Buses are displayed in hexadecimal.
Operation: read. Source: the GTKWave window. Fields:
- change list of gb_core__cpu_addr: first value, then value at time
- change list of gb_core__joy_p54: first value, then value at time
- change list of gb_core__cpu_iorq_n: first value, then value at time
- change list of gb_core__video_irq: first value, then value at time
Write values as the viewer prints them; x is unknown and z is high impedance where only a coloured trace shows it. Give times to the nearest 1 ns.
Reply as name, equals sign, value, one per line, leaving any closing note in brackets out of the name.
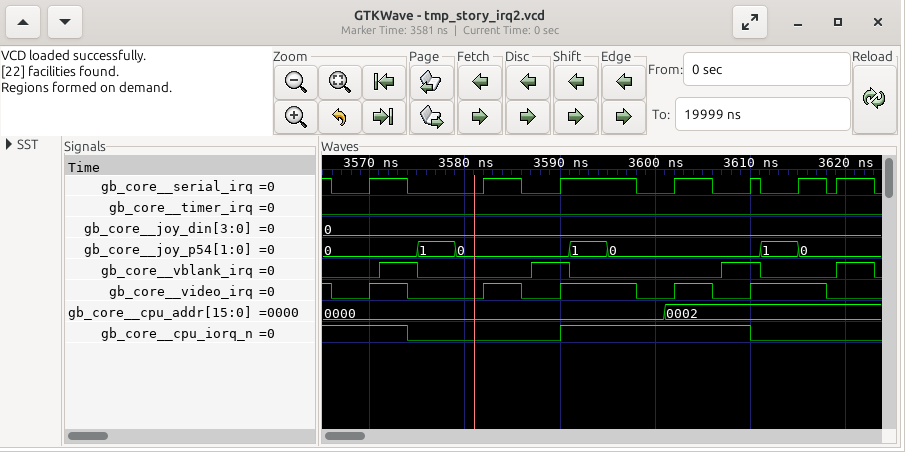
change list of gb_core__cpu_addr: first value, then value at time = 0000, 0002 at 3601 ns
change list of gb_core__joy_p54: first value, then value at time = 0, 1 at 3575 ns, 0 at 3579 ns, 1 at 3591 ns, 0 at 3595 ns, 1 at 3611 ns, 0 at 3615 ns
change list of gb_core__cpu_iorq_n: first value, then value at time = 1, 0 at 3574 ns, 1 at 3590 ns, 0 at 3610 ns
change list of gb_core__video_irq: first value, then value at time = 1, 0 at 3566 ns, 1 at 3570 ns, 0 at 3574 ns, 1 at 3582 ns, 0 at 3586 ns, 1 at 3590 ns, 0 at 3598 ns, 1 at 3602 ns, 0 at 3606 ns, 1 at 3610 ns, 0 at 3618 ns
